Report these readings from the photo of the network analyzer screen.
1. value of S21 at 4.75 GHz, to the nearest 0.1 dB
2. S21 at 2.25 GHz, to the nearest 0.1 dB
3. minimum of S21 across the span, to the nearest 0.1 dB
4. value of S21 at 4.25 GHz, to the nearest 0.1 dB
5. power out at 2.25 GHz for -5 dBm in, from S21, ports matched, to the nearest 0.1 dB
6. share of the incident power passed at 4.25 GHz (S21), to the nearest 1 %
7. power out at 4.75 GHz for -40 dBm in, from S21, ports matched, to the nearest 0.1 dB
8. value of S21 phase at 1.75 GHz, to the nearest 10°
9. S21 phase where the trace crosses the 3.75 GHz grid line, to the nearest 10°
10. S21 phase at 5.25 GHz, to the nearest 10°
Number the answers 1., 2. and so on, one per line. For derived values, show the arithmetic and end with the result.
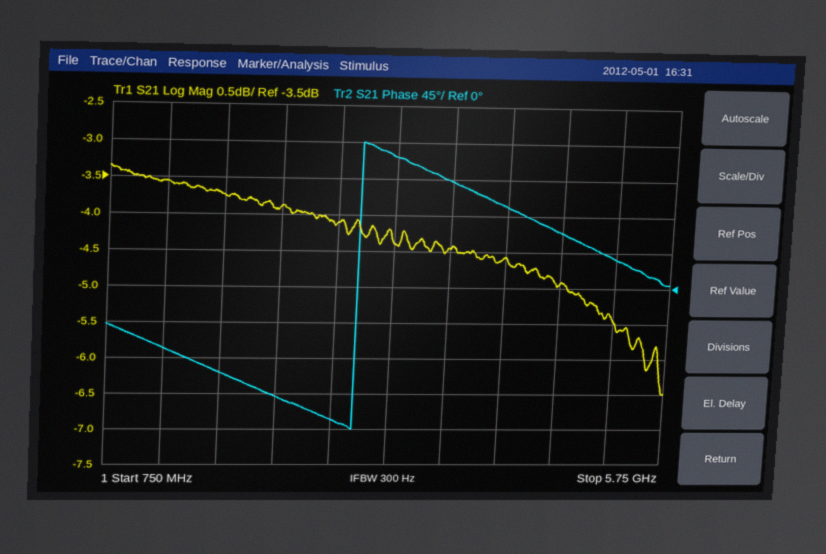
1. -4.9 dB
2. -3.9 dB
3. -6.5 dB
4. -4.6 dB
5. -5 dBm + (-3.9 dB) = -8.9 dBm
6. 10^(-4.6/10) ≈ 35 %
7. -40 dBm + (-4.9 dB) = -44.9 dBm
8. -110°
9. 130°
10. 40°
